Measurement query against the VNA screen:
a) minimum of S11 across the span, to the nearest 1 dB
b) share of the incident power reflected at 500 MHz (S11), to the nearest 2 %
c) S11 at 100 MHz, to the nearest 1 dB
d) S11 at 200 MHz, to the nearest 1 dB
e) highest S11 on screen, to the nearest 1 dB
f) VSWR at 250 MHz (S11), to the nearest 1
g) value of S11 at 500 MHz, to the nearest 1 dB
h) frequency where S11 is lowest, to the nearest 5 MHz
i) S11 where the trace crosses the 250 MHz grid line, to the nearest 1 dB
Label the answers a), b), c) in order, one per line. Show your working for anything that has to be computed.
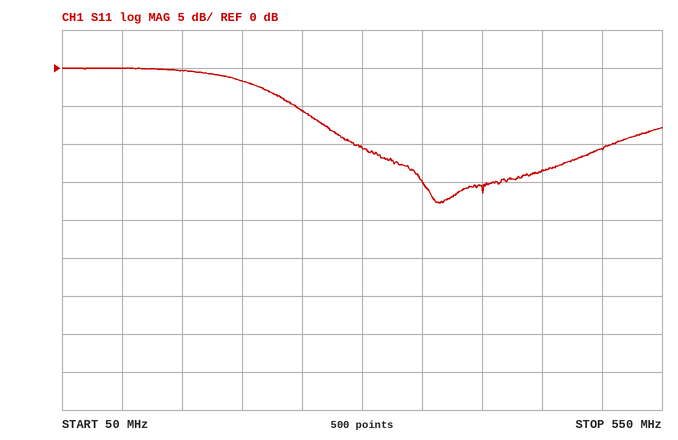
a) -18 dB
b) 10^(-11/10) ≈ 8 %
c) 0 dB
d) -2 dB
e) 0 dB
f) |Γ| = 10^(-6/20) = 0.5012; VSWR = (1 + 0.5012)/(1 − 0.5012) ≈ 3
g) -11 dB
h) 365 MHz
i) -6 dB
